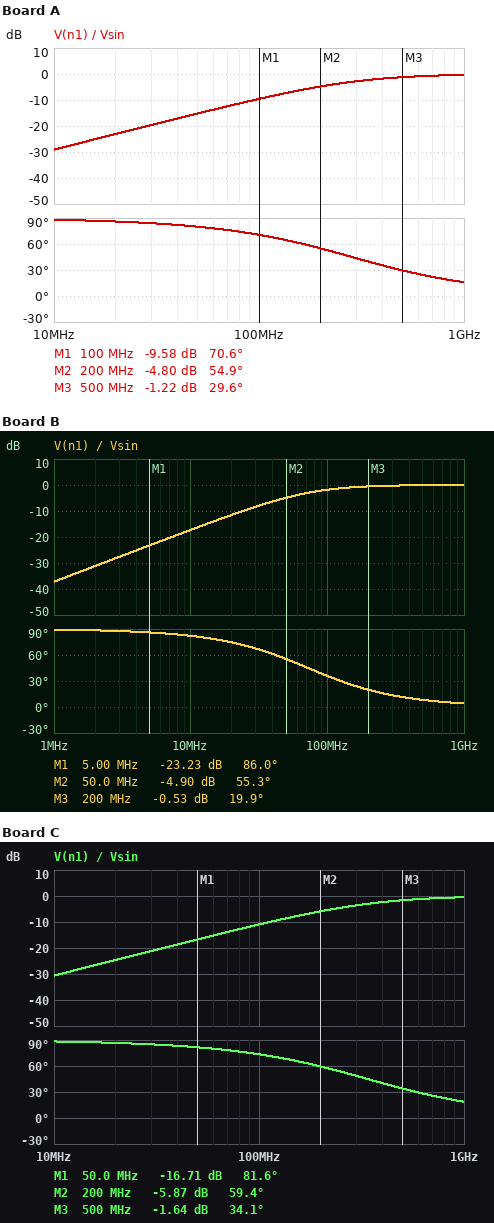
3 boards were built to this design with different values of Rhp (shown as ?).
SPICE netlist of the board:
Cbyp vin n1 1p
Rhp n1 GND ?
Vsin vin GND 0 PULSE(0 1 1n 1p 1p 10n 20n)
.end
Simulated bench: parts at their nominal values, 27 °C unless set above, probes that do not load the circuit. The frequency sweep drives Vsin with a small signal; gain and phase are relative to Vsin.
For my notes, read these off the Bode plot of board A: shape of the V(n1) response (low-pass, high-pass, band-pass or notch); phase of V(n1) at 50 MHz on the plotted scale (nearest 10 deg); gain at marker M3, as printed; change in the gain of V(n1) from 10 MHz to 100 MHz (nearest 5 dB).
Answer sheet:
high-pass
80 deg
-1.22 dB
20 dB
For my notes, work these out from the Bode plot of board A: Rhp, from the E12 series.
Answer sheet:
560 Ω
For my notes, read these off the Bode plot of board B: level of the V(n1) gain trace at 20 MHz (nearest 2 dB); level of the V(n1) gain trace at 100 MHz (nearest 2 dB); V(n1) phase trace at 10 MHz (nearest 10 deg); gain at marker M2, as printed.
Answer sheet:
-12 dB
-2 dB
80 deg
-4.90 dB
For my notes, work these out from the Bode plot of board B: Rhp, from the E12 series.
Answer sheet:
2.2 kΩ
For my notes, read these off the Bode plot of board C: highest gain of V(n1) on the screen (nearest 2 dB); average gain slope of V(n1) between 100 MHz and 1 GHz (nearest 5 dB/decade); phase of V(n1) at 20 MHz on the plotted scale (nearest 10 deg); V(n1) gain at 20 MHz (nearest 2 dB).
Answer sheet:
0 dB
10 dB/decade
90 deg
-24 dB
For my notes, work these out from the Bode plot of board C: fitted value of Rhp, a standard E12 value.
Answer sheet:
470 Ω
